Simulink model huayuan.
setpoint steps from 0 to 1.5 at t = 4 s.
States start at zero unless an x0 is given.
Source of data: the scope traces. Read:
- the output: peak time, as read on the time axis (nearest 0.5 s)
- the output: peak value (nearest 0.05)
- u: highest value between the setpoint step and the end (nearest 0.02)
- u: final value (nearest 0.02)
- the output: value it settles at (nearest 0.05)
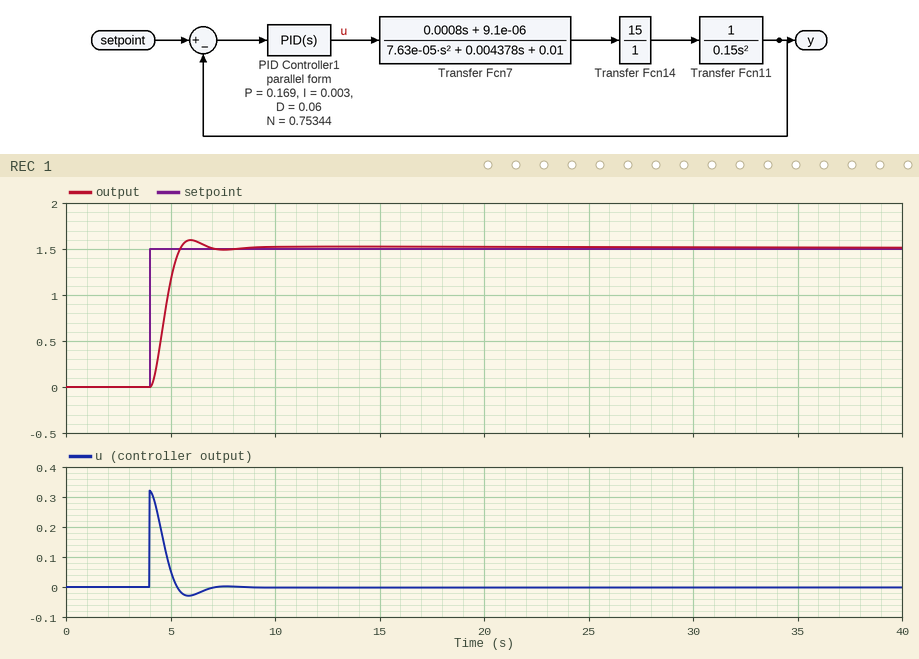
6.0 s
1.60
0.32
0.00
1.50
